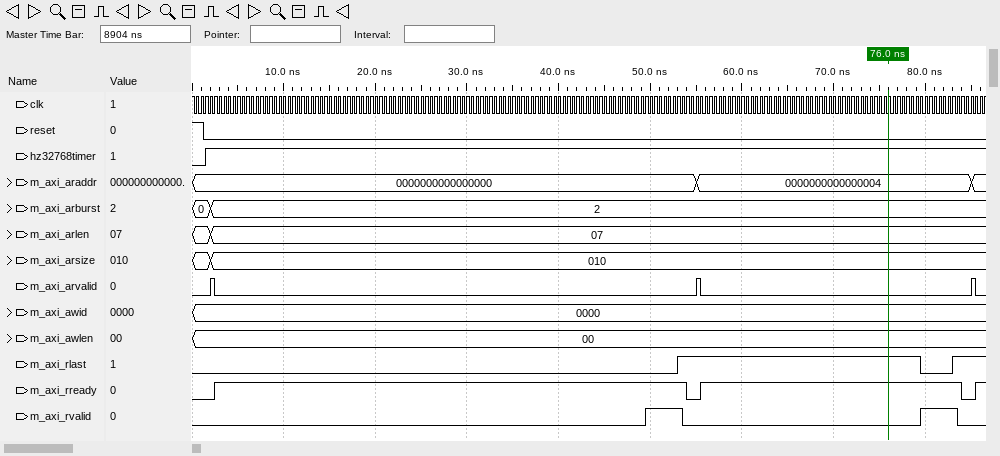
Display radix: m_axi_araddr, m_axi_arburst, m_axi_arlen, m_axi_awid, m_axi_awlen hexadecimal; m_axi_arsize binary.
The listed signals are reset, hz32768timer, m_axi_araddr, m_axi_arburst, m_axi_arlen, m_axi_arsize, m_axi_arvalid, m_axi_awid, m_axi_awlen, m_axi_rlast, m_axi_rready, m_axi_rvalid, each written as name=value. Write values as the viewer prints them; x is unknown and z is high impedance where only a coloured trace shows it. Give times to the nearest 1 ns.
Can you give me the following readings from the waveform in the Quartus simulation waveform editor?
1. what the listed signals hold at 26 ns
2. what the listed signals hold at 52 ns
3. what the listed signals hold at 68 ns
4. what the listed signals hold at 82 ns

reset=0, hz32768timer=1, m_axi_araddr=0000000000000000, m_axi_arburst=2, m_axi_arlen=07, m_axi_arsize=010, m_axi_arvalid=0, m_axi_awid=0000, m_axi_awlen=00, m_axi_rlast=0, m_axi_rready=1, m_axi_rvalid=0
reset=0, hz32768timer=1, m_axi_araddr=0000000000000000, m_axi_arburst=2, m_axi_arlen=07, m_axi_arsize=010, m_axi_arvalid=0, m_axi_awid=0000, m_axi_awlen=00, m_axi_rlast=0, m_axi_rready=1, m_axi_rvalid=1
reset=0, hz32768timer=1, m_axi_araddr=0000000000000004, m_axi_arburst=2, m_axi_arlen=07, m_axi_arsize=010, m_axi_arvalid=0, m_axi_awid=0000, m_axi_awlen=00, m_axi_rlast=1, m_axi_rready=1, m_axi_rvalid=0
reset=0, hz32768timer=1, m_axi_araddr=0000000000000004, m_axi_arburst=2, m_axi_arlen=07, m_axi_arsize=010, m_axi_arvalid=0, m_axi_awid=0000, m_axi_awlen=00, m_axi_rlast=0, m_axi_rready=1, m_axi_rvalid=1
